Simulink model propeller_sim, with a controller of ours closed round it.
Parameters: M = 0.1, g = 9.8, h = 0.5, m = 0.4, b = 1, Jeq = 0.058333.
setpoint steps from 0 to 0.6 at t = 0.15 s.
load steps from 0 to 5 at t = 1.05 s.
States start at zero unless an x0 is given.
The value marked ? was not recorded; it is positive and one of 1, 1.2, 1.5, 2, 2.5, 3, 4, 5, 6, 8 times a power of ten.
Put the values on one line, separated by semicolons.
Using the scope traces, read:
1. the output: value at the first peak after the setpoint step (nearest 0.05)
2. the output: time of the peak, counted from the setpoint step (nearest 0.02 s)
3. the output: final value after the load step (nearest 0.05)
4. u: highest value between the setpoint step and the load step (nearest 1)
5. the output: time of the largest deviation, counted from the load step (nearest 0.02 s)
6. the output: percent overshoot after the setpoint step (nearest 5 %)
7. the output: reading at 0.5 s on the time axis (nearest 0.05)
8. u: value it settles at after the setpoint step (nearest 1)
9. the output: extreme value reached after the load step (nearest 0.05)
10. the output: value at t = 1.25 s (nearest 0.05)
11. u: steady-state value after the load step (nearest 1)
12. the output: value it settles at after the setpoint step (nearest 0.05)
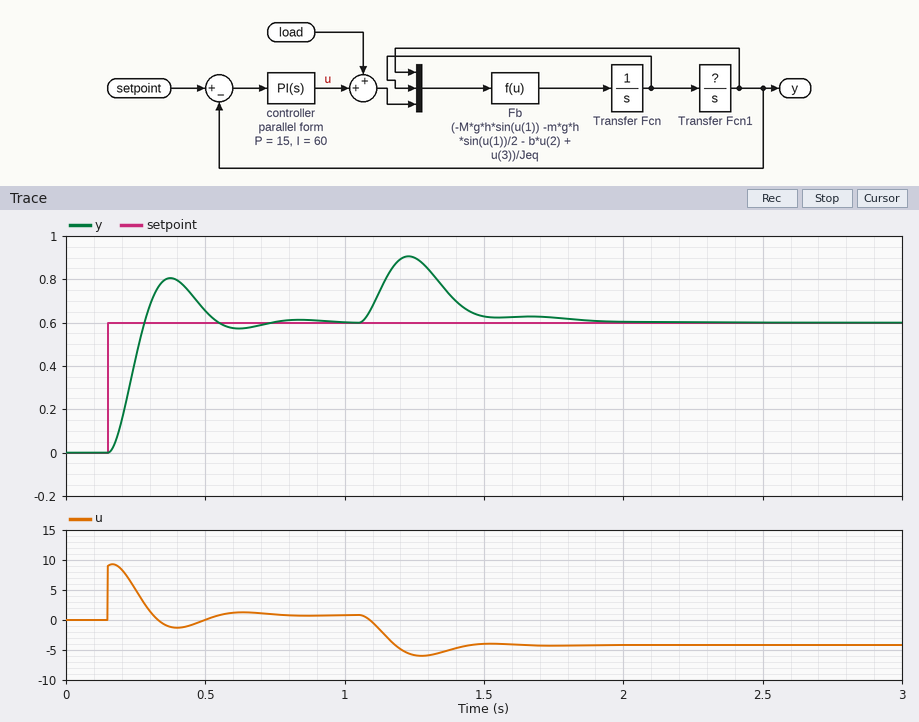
0.80; 0.22 s; 0.60; 9; 0.18 s; 35 %; 0.65; 1; 0.90; 0.90; -4; 0.60
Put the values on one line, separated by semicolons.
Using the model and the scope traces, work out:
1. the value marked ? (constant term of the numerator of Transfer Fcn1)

1
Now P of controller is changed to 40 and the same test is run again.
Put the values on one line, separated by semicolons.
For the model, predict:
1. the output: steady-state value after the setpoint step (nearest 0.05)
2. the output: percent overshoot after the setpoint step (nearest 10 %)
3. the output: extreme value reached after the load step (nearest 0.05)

0.60; 40 %; 0.75
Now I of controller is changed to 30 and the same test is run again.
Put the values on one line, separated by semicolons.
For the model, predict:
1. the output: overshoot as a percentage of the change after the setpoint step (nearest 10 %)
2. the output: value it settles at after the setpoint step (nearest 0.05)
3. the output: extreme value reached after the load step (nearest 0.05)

20 %; 0.60; 0.95
